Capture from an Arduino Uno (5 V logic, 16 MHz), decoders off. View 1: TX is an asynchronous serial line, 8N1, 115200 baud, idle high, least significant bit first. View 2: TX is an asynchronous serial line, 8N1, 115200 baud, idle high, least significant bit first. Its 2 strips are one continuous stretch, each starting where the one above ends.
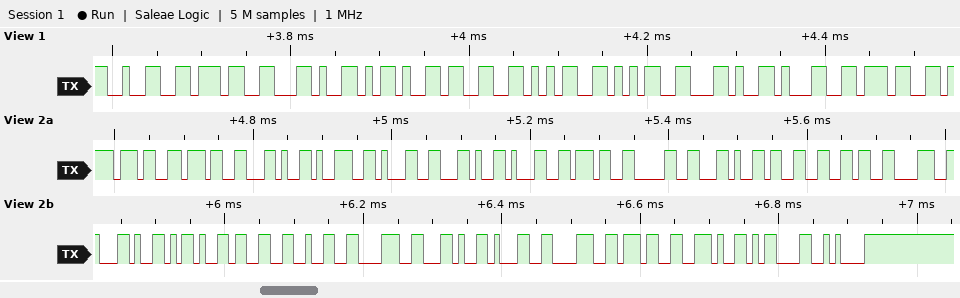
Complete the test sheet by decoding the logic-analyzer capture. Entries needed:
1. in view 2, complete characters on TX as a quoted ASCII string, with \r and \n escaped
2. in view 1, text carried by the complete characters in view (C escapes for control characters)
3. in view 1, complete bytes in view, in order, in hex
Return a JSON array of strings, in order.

["\"77,91,170,368,-328,187.\\r\\n\"", "\"27,-355,17\"", "32 37 2C 2D 33 35 35 2C 31 37"]
